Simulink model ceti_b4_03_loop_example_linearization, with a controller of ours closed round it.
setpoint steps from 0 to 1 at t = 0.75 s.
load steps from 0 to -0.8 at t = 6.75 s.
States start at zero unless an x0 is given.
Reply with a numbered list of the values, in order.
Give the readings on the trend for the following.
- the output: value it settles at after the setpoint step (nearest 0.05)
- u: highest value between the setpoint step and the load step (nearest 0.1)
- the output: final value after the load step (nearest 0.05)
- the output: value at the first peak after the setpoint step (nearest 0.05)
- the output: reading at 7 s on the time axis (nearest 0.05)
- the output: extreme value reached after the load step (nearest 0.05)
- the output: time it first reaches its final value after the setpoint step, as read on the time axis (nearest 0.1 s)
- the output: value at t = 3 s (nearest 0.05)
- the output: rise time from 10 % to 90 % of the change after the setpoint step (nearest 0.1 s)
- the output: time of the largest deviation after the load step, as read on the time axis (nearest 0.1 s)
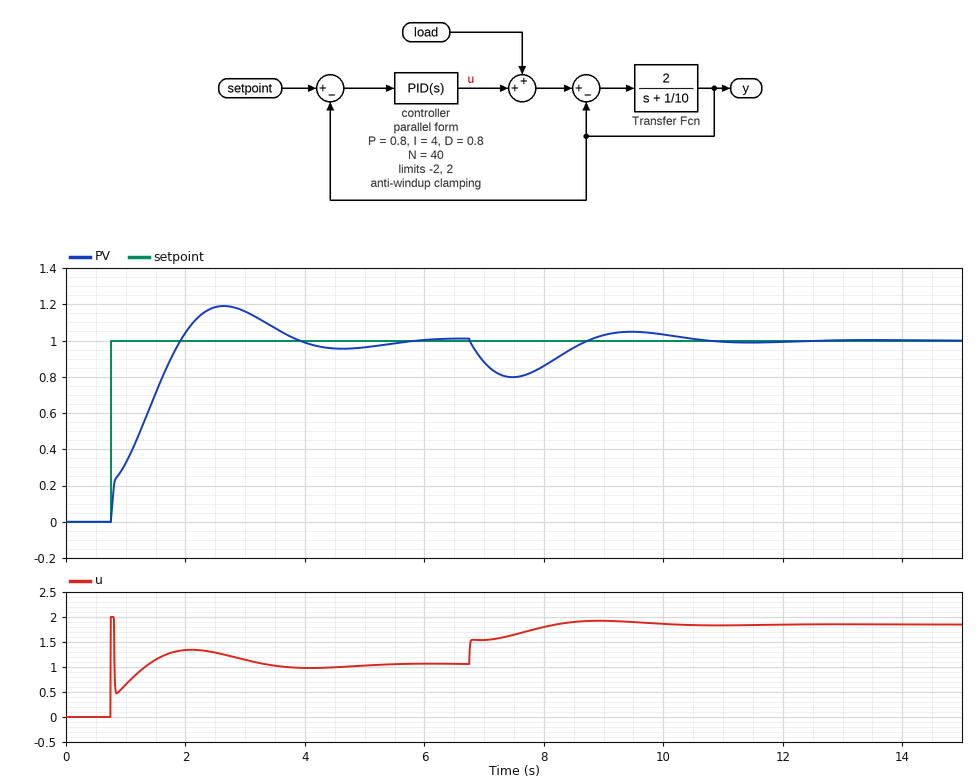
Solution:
1. 1.00
2. 2.0
3. 1.00
4. 1.20
5. 0.90
6. 0.80
7. 1.9 s
8. 1.15
9. 1.0 s
10. 7.5 s
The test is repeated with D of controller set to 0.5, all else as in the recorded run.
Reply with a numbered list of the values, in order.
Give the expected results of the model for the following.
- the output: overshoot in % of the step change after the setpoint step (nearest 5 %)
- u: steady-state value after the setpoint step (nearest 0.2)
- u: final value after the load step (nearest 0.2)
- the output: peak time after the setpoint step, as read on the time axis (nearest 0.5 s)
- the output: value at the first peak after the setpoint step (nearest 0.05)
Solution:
1. 15 %
2. 1.0
3. 1.8
4. 2.5 s
5. 1.15
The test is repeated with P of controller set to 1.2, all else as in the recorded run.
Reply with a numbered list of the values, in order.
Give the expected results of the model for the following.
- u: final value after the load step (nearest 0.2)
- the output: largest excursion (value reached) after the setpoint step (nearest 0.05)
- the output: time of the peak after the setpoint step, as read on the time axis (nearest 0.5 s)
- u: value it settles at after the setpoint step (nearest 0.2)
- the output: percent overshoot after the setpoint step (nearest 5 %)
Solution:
1. 1.8
2. 1.15
3. 2.5 s
4. 1.0
5. 15 %
